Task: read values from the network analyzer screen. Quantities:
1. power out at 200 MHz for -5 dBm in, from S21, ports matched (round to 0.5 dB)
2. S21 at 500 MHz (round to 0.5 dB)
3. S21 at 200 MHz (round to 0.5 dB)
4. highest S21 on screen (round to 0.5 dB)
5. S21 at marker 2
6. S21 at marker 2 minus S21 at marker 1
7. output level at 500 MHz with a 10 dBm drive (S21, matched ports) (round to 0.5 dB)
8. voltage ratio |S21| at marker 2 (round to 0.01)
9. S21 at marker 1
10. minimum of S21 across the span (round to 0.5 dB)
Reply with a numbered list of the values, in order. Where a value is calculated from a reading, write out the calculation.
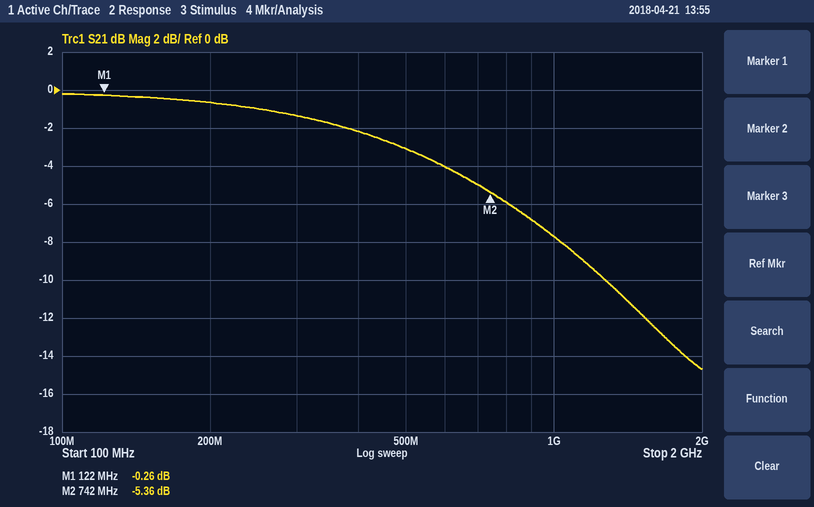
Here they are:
1. -5 dBm + (-0.5 dB) = -5.5 dBm
2. -3.0 dB
3. -0.5 dB
4. 0.0 dB
5. -5.36 dB
6. -5.36 − (-0.26) = -5.10 dB
7. 10 dBm + (-3.0 dB) = 7.0 dBm
8. 10^(-5.36/20) ≈ 0.54
9. -0.26 dB
10. -14.5 dB
